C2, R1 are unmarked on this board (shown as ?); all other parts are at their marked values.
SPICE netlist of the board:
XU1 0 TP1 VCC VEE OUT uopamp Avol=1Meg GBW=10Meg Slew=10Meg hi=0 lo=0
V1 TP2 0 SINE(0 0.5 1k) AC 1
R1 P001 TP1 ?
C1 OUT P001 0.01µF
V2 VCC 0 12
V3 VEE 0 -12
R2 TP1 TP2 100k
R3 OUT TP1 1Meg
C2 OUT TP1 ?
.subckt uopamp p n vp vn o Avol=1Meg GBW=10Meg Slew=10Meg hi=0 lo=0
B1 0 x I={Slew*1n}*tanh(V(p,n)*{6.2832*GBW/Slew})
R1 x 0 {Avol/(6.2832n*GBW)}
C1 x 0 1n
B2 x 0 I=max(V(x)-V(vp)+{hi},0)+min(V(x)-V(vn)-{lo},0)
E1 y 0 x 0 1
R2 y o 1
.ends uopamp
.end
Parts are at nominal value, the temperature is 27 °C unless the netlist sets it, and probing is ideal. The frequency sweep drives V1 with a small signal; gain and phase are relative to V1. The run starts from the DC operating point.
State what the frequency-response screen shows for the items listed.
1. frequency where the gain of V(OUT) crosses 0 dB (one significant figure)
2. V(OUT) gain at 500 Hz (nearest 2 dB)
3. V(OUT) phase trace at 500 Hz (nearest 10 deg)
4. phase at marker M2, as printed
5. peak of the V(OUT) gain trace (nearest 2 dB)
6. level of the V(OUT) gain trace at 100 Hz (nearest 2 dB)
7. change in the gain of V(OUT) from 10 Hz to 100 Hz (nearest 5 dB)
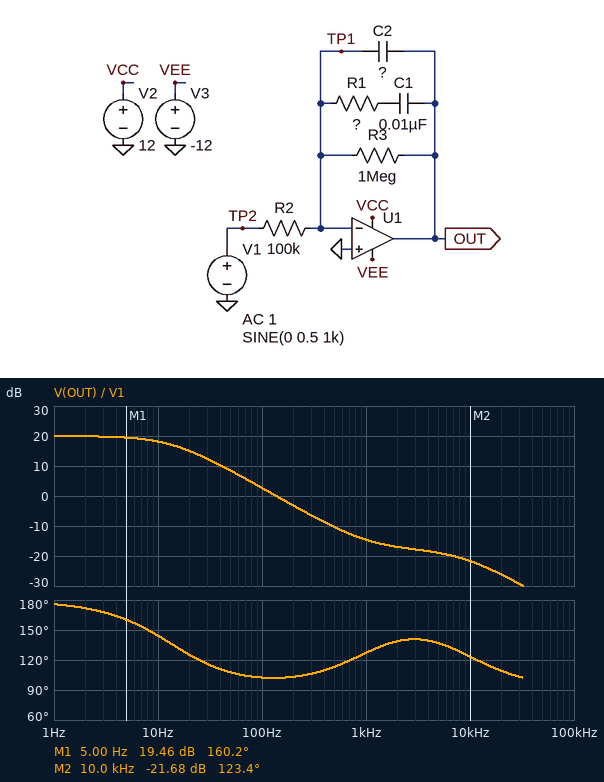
100 Hz
-10 dB
110 deg
123.4 deg
20 dB
2 dB
-15 dB
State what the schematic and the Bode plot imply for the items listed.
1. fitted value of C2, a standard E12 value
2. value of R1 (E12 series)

1.5 nF
15 kΩ
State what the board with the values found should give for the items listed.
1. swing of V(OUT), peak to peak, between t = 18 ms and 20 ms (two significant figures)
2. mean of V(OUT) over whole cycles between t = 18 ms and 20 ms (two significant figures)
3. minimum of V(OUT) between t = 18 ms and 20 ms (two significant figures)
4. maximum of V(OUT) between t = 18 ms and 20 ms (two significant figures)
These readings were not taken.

190 mV
-13 mV
-110 mV
81 mV
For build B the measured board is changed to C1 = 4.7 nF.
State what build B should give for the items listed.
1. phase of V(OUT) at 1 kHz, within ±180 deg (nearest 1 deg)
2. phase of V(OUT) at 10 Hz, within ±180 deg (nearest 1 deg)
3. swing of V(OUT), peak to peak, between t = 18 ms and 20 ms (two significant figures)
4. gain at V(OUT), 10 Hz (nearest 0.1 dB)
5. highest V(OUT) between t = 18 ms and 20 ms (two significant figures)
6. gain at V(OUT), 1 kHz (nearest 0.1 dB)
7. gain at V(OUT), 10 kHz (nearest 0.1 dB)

109 deg
159 deg
280 mV
19.4 dB
130 mV
-11.2 dB
-22.0 dB
